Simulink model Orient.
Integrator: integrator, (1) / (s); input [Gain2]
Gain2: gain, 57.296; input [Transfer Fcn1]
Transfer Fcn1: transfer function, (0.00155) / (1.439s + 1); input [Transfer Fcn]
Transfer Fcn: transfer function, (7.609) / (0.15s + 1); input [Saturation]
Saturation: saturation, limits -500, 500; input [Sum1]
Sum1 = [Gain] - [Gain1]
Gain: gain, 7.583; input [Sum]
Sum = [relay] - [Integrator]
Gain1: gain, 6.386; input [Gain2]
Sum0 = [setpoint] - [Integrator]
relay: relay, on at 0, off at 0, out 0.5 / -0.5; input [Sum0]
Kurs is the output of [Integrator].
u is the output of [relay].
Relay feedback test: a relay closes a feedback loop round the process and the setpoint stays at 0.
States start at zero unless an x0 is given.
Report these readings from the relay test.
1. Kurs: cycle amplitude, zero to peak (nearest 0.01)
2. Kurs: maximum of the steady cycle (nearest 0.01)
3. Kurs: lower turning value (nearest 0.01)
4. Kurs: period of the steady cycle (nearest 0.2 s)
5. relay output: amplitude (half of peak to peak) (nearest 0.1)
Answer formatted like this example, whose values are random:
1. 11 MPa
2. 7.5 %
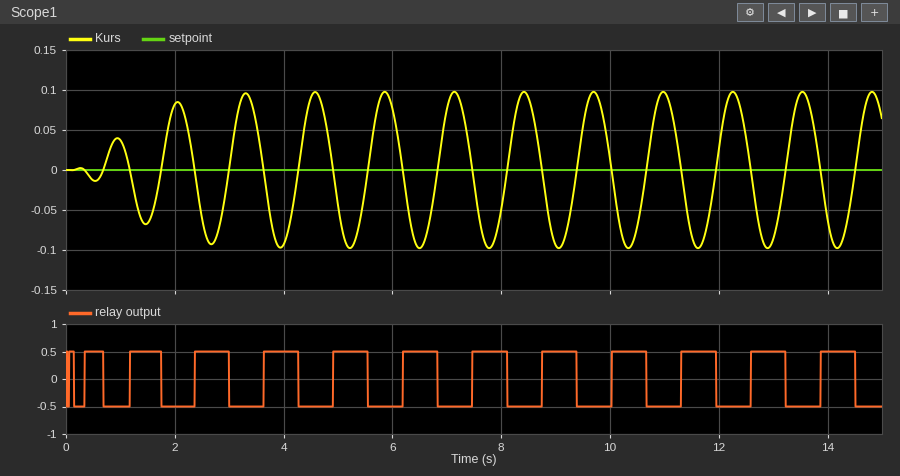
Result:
1. 0.10
2. 0.10
3. -0.10
4. 1.2 s
5. 0.5
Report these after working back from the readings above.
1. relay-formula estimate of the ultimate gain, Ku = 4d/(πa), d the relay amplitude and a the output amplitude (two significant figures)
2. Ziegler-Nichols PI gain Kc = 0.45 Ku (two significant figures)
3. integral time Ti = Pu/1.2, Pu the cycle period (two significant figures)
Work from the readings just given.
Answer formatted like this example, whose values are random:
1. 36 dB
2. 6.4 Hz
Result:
1. 6.4
2. 2.9
3. 1.0 s
